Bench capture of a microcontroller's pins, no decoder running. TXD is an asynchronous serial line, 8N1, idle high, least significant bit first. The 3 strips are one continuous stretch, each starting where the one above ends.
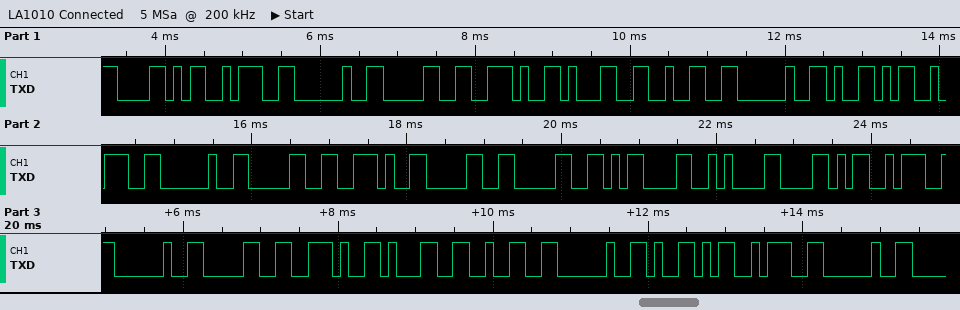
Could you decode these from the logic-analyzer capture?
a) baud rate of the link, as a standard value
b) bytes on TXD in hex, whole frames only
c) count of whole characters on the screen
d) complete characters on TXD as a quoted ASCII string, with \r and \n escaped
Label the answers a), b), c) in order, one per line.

a) 9600 baud
b) 58 3A 20 30 2E 31 32 20 59 3A 20 30 2E 30 30 0D 0A 58 3A 20 30 2E 31 32 20 59 3A 20
c) 28
d) "X: 0.12 Y: 0.00\r\nX: 0.12 Y: "
